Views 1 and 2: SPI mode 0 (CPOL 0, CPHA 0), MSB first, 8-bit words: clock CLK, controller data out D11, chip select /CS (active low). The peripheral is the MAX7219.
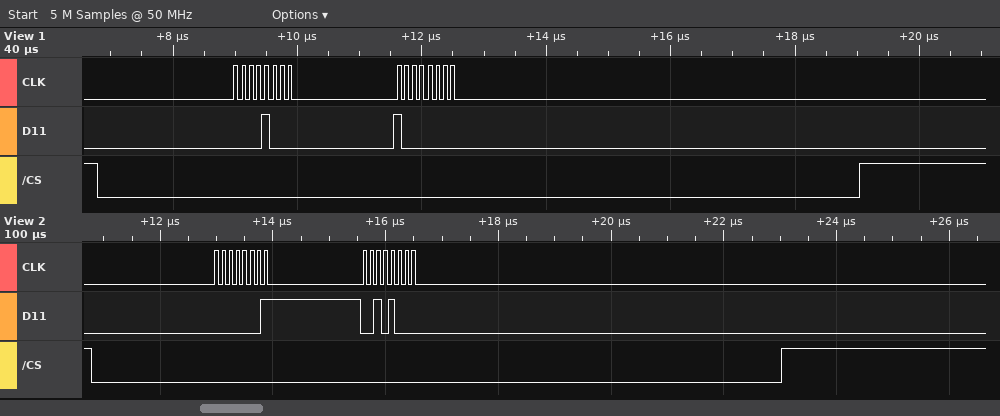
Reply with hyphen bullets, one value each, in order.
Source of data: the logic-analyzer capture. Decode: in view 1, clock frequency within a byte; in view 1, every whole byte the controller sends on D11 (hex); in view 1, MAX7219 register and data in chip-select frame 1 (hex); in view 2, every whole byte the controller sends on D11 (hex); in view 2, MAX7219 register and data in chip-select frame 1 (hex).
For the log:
- 8 MHz
- 08 80
- register 0x8, data 0x80
- 01 28
- register 0x1, data 0x28
